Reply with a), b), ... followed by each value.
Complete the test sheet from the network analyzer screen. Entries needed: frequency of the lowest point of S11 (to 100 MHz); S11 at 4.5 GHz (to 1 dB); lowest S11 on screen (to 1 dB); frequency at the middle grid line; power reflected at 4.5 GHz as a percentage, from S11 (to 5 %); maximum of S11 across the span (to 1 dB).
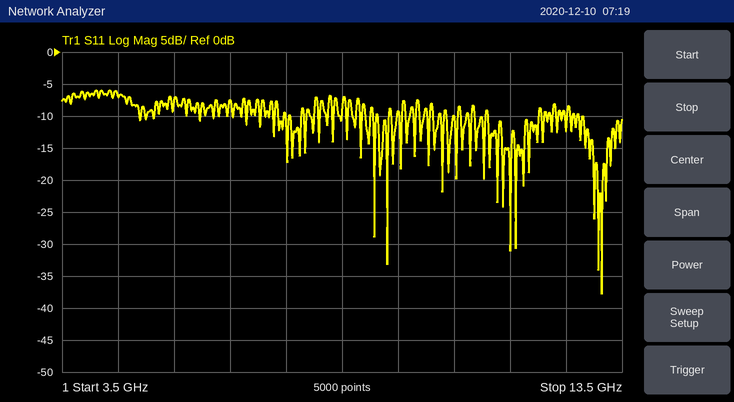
a) 13.1 GHz
b) -7 dB
c) -38 dB
d) 8.5 GHz
e) 20 %
f) -6 dB
